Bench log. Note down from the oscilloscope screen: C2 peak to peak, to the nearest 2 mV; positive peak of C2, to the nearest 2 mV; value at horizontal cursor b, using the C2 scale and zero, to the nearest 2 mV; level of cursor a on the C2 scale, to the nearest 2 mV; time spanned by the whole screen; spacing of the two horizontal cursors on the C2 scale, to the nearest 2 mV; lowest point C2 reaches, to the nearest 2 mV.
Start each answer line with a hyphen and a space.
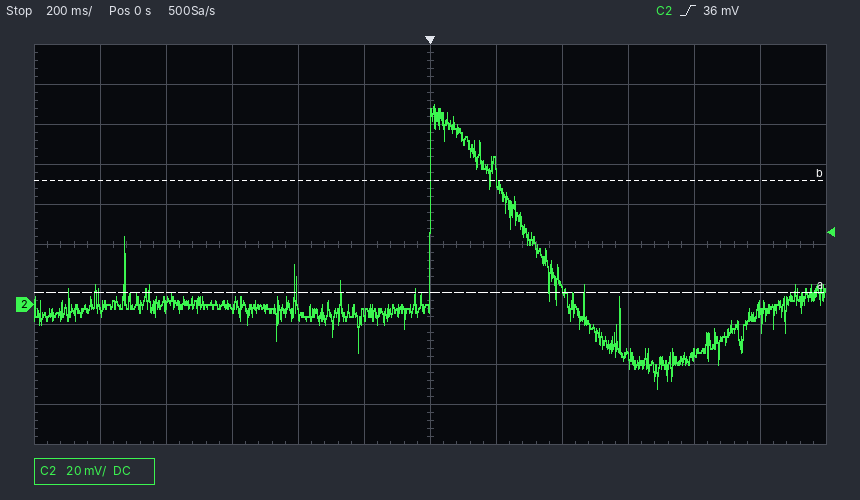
- 142 mV
- 100 mV
- 62 mV
- 6 mV
- 2.4 s
- 56 mV
- -42 mV
